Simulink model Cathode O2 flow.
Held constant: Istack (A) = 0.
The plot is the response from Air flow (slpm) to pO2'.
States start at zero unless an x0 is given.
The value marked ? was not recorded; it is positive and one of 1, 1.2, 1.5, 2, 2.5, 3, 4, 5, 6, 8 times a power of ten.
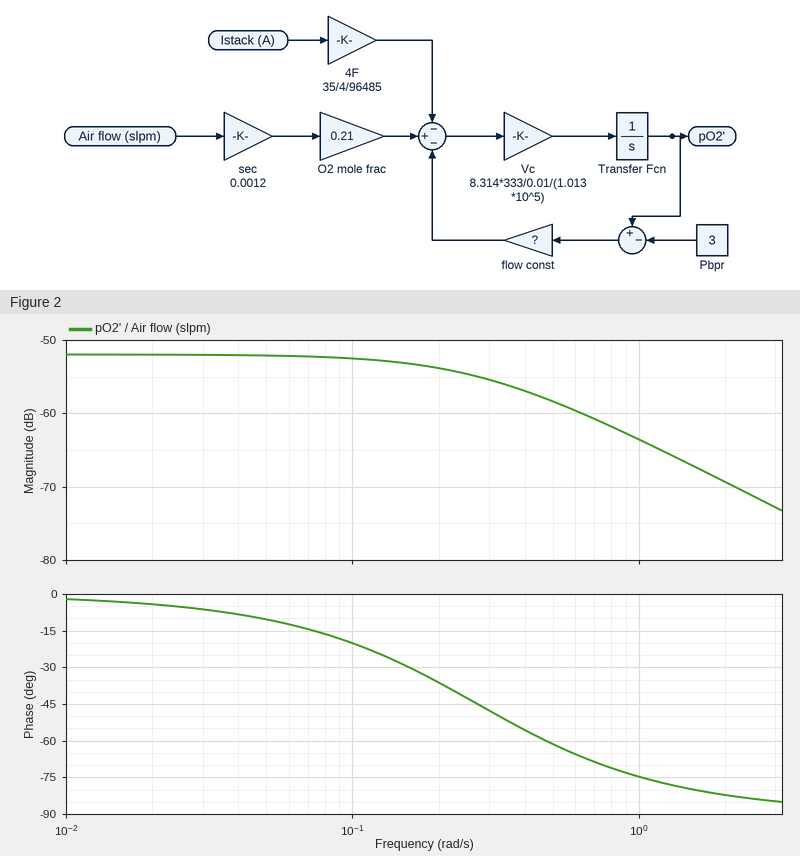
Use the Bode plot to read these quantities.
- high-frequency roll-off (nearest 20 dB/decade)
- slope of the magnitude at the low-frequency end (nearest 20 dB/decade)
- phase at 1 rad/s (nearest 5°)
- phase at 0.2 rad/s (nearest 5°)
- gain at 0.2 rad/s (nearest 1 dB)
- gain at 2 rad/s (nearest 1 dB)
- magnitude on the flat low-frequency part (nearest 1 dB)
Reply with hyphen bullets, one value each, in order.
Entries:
- -20 dB/decade
- 0 dB/decade
- -75°
- -35°
- -54 dB
- -69 dB
- -52 dB
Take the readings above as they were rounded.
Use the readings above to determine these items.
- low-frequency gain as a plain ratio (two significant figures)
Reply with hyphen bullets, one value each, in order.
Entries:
- 0.0025
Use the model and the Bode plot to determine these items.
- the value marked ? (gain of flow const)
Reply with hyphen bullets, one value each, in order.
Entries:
- 0.1
